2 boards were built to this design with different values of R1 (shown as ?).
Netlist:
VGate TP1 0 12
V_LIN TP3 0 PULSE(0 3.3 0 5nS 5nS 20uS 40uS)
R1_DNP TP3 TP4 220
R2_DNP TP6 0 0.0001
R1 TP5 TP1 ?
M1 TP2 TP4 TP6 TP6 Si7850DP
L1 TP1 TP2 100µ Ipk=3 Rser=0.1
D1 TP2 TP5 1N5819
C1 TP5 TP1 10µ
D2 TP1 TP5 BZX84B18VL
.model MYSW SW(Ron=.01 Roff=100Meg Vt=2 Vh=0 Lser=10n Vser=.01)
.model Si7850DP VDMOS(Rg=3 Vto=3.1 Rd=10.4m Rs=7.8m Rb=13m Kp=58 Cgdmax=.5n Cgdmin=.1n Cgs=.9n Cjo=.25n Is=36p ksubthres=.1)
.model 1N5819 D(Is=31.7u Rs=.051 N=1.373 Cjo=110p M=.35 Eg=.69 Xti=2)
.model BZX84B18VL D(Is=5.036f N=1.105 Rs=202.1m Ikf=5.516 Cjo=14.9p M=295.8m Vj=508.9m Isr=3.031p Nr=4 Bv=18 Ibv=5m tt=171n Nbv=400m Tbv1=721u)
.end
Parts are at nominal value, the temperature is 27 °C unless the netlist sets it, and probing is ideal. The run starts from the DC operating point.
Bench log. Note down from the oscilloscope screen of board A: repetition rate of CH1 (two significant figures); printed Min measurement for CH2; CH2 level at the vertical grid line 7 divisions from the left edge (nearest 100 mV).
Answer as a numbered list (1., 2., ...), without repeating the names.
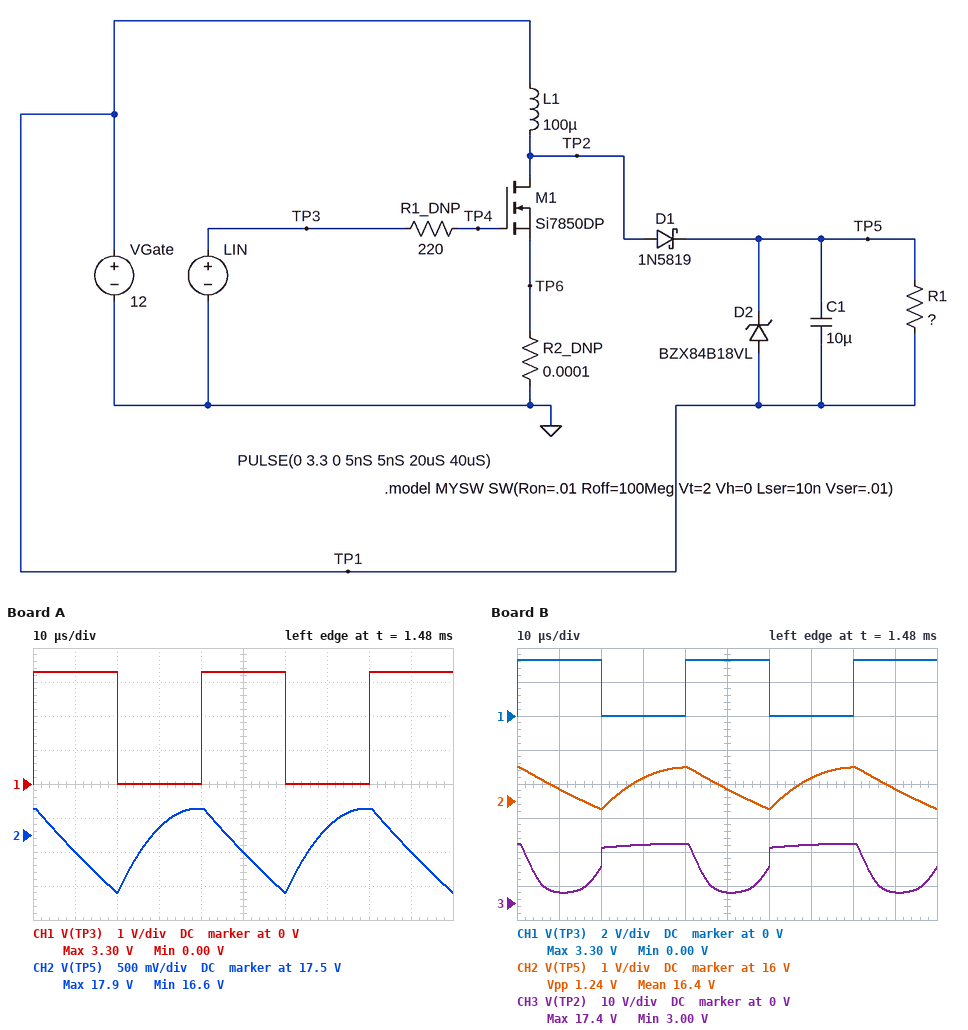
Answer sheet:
1. 25 kHz
2. 16.6 V
3. 17.6 V
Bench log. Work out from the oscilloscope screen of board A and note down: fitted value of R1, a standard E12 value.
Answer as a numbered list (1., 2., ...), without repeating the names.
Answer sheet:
1. 8.2 Ω
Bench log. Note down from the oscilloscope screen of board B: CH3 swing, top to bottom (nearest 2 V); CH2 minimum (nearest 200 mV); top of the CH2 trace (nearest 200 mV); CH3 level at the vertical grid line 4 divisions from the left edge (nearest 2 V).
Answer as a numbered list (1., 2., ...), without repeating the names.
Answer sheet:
1. 14 V
2. 15.8 V
3. 17.0 V
4. 18 V
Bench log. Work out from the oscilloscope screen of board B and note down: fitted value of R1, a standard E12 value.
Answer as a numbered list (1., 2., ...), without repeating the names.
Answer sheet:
1. 6.8 Ω
